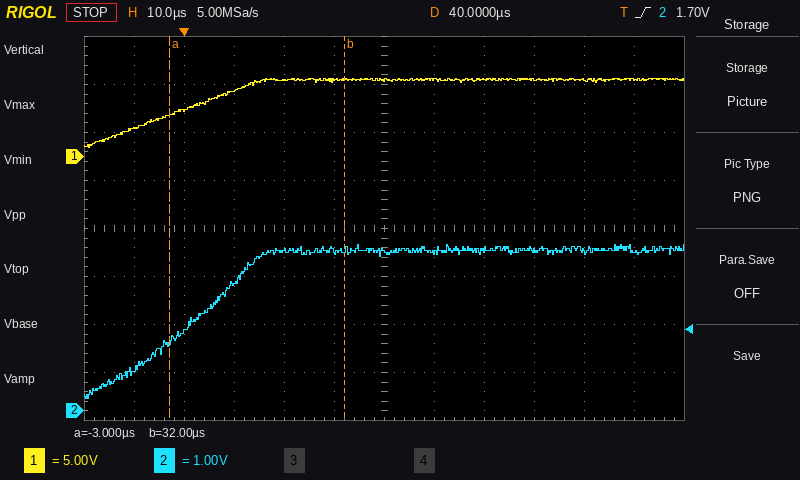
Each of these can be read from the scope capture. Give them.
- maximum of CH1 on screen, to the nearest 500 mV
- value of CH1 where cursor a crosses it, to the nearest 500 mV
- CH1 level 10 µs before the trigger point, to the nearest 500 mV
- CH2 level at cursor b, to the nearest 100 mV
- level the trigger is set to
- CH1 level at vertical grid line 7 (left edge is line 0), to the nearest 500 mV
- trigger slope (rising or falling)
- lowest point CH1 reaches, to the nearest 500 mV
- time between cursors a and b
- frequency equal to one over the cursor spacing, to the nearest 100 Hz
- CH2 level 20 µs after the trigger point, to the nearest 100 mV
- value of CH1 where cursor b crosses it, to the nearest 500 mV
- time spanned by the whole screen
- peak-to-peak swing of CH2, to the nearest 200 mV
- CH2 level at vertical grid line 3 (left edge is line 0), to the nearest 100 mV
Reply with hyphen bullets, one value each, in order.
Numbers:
- 8.0 V
- 4.5 V
- 3.0 V
- 3.3 V
- 1.70 V
- 8.0 V
- rising
- 1.0 V
- 35 µs
- 28.6 kHz
- 3.3 V
- 8.0 V
- 120 µs
- 3.2 V
- 2.7 V
